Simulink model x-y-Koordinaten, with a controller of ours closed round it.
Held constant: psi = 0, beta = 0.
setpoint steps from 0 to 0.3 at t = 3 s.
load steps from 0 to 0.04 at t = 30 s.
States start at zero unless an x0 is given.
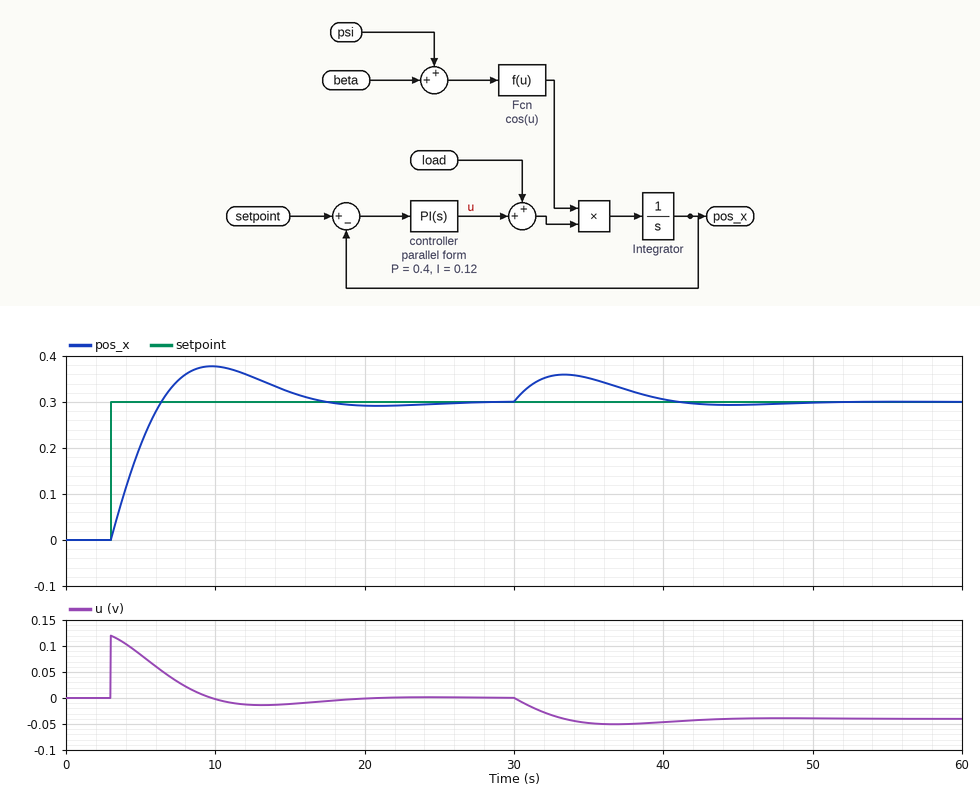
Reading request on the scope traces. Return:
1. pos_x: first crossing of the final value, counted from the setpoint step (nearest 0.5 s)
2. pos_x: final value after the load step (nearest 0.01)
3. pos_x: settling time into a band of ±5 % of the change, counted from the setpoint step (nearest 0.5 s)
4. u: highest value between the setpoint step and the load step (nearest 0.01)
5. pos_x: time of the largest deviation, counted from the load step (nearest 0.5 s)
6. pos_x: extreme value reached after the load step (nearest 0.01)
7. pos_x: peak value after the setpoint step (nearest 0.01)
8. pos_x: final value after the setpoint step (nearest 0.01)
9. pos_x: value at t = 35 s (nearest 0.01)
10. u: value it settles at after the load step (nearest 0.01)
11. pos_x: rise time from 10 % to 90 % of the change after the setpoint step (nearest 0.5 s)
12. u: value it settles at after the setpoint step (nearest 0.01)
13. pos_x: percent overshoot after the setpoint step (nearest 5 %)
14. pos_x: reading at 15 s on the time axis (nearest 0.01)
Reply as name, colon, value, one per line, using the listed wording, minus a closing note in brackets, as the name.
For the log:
pos_x: first crossing of the final value, counted from the setpoint step: 3.5 s
pos_x: final value after the load step: 0.30
pos_x: settling time into a band of ±5 % of the change, counted from the setpoint step: 12.5 s
u: highest value between the setpoint step and the load step: 0.12
pos_x: time of the largest deviation, counted from the load step: 3.5 s
pos_x: extreme value reached after the load step: 0.36
pos_x: peak value after the setpoint step: 0.38
pos_x: final value after the setpoint step: 0.30
pos_x: value at t = 35 s: 0.35
u: value it settles at after the load step: -0.04
pos_x: rise time from 10 % to 90 % of the change after the setpoint step: 2.5 s
u: value it settles at after the setpoint step: 0.00
pos_x: percent overshoot after the setpoint step: 25 %
pos_x: reading at 15 s on the time axis: 0.32
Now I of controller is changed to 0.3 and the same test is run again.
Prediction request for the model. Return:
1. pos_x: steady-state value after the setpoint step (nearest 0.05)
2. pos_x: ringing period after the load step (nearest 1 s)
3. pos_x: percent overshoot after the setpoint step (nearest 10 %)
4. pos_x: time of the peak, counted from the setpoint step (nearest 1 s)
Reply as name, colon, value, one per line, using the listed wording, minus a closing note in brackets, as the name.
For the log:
pos_x: steady-state value after the setpoint step: 0.30
pos_x: ringing period after the load step: 12 s
pos_x: percent overshoot after the setpoint step: 40 %
pos_x: time of the peak, counted from the setpoint step: 5 s
